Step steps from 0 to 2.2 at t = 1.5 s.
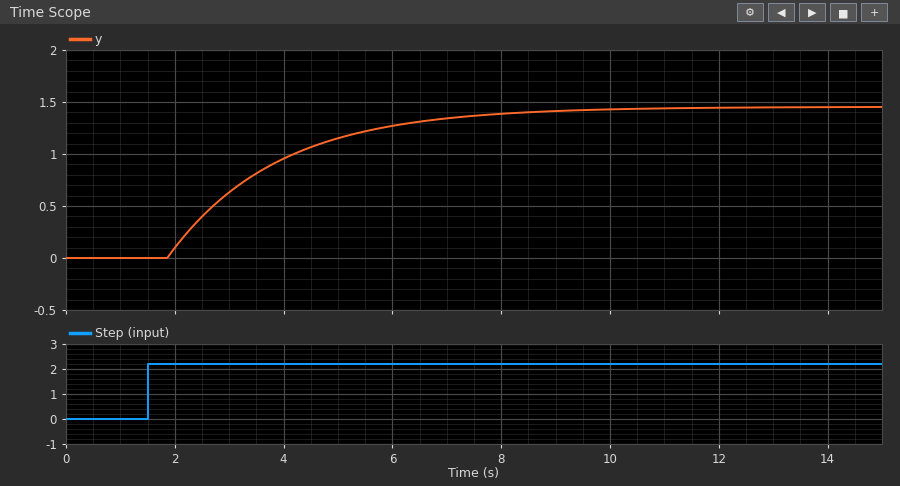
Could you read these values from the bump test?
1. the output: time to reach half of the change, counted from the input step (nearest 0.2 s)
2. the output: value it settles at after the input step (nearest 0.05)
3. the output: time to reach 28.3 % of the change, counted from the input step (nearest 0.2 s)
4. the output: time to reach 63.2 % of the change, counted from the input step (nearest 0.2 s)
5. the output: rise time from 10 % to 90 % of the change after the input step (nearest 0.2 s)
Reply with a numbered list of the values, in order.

1. 1.8 s
2. 1.45
3. 1.0 s
4. 2.4 s
5. 4.4 s
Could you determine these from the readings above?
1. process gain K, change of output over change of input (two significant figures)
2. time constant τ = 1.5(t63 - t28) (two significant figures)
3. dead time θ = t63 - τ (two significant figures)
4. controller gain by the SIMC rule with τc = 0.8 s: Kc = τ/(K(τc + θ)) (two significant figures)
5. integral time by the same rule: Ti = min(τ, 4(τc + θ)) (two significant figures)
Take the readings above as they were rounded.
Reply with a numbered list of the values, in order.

1. 0.66
2. 2.1 s
3. 0.30 s
4. 2.9
5. 2.1 s
